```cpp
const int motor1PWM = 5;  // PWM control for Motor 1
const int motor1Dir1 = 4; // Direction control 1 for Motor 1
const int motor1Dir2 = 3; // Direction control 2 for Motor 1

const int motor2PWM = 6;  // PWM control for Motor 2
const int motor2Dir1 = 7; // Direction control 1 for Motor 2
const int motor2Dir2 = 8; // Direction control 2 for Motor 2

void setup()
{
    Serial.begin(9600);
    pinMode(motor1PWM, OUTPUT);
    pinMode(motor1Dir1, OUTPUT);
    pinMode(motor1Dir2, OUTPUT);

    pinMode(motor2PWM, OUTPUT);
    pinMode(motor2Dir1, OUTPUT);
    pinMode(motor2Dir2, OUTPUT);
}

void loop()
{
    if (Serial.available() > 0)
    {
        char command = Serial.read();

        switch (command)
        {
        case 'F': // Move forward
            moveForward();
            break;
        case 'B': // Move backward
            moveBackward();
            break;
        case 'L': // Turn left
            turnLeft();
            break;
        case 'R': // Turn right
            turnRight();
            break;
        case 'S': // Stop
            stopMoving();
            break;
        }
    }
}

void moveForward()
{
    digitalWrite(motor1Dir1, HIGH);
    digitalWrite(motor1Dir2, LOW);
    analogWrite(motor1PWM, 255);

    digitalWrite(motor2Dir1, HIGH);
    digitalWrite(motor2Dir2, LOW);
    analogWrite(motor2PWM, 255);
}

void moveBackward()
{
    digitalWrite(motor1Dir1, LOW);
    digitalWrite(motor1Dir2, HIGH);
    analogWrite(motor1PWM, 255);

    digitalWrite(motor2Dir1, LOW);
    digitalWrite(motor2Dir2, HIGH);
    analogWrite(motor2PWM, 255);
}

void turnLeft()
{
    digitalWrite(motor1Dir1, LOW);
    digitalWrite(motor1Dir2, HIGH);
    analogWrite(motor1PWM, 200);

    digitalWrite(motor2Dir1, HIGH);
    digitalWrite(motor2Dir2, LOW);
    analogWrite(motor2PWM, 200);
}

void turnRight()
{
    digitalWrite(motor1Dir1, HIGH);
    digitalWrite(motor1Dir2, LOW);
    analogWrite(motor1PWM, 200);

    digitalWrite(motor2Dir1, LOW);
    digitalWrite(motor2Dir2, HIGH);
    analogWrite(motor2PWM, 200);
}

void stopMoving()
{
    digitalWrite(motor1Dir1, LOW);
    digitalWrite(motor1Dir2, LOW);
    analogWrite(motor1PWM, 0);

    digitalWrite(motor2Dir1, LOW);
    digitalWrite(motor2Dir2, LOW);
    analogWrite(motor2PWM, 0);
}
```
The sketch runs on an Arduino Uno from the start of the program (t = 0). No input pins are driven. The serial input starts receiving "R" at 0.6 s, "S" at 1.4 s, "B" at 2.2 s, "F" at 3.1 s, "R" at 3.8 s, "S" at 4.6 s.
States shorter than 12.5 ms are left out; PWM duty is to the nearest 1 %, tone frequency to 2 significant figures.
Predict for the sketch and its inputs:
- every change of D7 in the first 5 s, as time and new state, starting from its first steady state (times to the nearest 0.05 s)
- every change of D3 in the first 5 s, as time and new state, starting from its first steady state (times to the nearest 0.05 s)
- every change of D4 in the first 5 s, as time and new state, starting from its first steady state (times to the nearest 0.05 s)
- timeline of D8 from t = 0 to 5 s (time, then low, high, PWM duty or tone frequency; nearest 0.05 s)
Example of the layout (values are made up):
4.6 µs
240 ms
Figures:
0 s low; 3.1 s high; 3.8 s low
0 s low; 2.2 s high; 3.1 s low
0 s low; 0.6 s high; 1.4 s low; 3.1 s high; 4.6 s low
0 s low; 0.6 s high; 1.4 s low; 2.2 s high; 3.1 s low; 3.8 s high; 4.6 s low
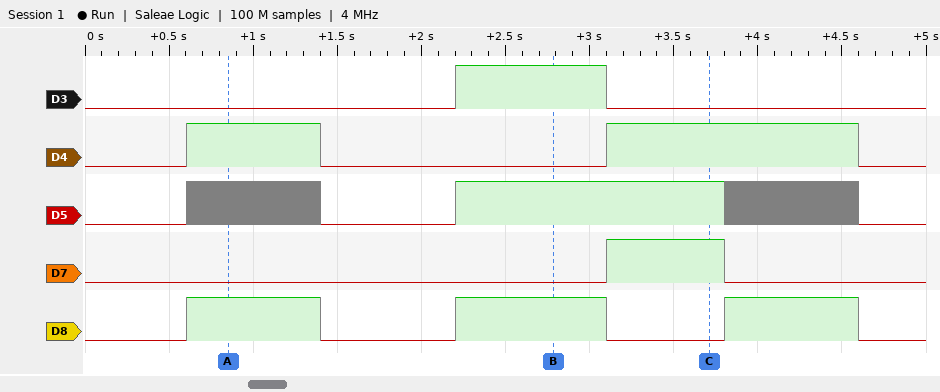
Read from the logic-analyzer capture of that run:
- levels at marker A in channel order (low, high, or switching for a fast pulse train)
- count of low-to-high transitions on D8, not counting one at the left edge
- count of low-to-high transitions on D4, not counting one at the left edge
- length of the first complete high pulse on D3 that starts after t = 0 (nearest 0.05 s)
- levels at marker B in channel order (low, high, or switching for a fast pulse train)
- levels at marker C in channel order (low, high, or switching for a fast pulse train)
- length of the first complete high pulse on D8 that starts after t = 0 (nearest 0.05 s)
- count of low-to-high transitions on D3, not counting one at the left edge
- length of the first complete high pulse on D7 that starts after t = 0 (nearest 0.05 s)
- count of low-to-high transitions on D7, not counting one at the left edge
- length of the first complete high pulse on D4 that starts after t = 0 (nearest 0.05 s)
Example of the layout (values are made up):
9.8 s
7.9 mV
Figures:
D3 low, D4 high, D5 switching, D7 low, D8 high
3
2
0.90 s
D3 high, D4 low, D5 high, D7 low, D8 high
D3 low, D4 high, D5 high, D7 high, D8 low
0.80 s
1
0.70 s
1
0.80 s
